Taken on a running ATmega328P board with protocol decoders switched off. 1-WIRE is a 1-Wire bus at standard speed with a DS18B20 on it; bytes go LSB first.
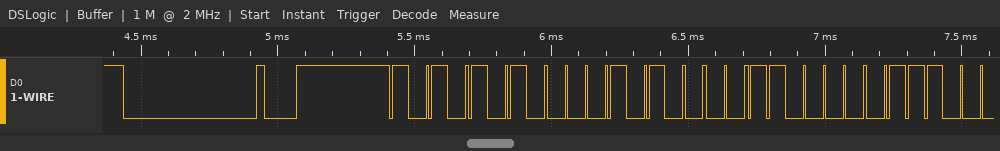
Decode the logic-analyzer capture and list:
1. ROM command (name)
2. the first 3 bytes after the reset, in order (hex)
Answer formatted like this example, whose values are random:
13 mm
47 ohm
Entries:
Match ROM
55 28 0C
